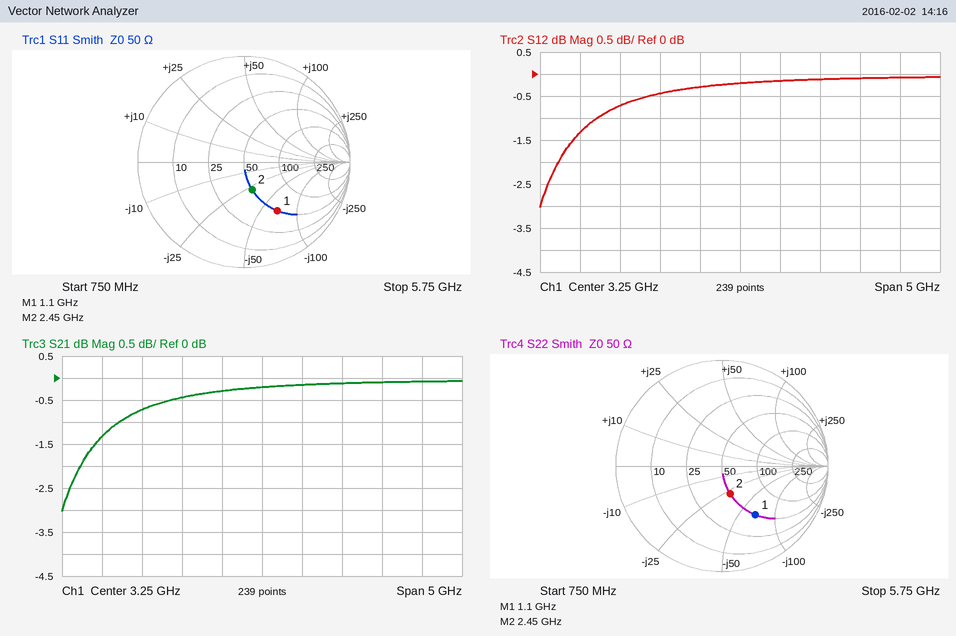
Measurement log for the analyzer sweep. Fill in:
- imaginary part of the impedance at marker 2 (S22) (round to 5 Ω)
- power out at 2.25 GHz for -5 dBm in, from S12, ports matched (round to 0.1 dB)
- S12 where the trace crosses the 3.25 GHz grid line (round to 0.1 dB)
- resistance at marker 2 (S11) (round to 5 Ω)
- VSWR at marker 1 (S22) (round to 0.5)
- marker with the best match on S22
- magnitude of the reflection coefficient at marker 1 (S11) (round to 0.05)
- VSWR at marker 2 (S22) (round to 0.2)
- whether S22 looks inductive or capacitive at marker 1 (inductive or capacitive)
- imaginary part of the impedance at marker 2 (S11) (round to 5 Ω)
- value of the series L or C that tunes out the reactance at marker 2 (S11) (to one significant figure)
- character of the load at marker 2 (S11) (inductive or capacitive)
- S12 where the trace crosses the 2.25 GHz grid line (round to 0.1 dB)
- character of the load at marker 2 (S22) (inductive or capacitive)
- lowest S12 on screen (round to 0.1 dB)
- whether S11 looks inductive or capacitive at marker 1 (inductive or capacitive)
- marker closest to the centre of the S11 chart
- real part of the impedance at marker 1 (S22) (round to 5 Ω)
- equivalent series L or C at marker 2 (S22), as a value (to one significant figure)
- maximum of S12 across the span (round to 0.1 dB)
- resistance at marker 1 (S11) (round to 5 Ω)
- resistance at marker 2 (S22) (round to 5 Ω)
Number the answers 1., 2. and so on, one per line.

1. -30 Ω
2. -5.4 dBm
3. -0.2 dB
4. 50 Ω
5. 3.5
6. marker 2
7. 0.55
8. 1.8
9. capacitive
10. -30 Ω
11. 2 nH
12. capacitive
13. -0.4 dB
14. capacitive
15. -3.0 dB
16. capacitive
17. marker 2
18. 50 Ω
19. 2 pF
20. -0.1 dB
21. 50 Ω
22. 50 Ω
